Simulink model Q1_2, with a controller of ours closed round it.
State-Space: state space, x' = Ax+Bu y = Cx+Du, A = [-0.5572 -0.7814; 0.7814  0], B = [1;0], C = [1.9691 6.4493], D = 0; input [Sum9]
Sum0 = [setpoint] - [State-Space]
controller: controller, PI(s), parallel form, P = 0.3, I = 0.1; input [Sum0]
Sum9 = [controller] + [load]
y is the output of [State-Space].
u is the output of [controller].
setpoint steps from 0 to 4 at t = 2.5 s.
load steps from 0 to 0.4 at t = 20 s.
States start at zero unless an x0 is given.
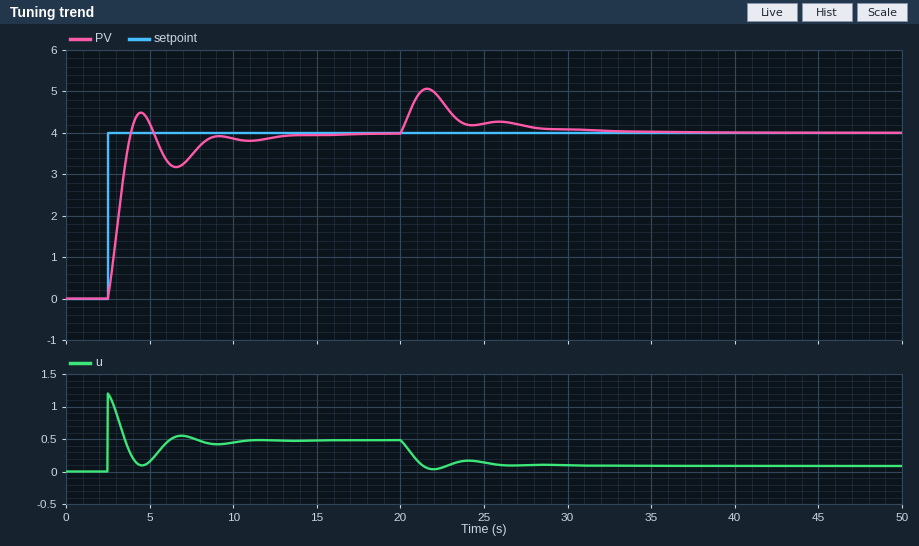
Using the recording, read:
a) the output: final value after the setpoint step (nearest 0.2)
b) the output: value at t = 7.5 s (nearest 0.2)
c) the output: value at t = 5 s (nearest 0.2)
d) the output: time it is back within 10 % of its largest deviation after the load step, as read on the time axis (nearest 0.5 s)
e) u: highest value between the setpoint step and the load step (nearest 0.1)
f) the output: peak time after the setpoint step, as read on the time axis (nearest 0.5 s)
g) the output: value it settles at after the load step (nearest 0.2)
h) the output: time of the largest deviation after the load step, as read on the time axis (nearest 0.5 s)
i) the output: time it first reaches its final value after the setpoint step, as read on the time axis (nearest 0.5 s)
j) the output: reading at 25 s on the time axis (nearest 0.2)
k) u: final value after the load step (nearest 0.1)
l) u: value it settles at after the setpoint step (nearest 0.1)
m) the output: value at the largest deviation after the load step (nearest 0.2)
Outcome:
4.0
3.4
4.2
28.5 s
1.2
4.5 s
4.0
21.5 s
4.0 s
4.2
0.1
0.5
5.0
